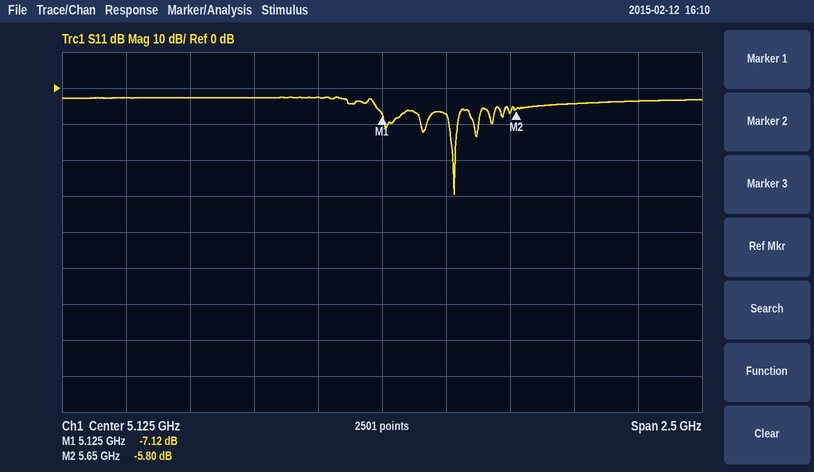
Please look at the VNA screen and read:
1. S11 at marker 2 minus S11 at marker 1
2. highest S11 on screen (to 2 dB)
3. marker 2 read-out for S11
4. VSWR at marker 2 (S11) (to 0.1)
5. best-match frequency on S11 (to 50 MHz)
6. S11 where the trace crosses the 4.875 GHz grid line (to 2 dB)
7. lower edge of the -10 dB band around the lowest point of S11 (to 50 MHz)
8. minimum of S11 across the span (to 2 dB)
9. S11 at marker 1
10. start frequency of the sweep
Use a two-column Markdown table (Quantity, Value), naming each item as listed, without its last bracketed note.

| Quantity | Value |
|---|---|
| S11 at marker 2 minus S11 at marker 1 | 1.32 dB |
| highest S11 on screen | -2 dB |
| marker 2 read-out for S11 | -5.80 dB |
| VSWR at marker 2 (S11) | 3.1 |
| best-match frequency on S11 | 5.40 GHz |
| S11 where the trace crosses the 4.875 GHz grid line | -2 dB |
| lower edge of the -10 dB band around the lowest point of S11 | 5.40 GHz |
| minimum of S11 across the span | -30 dB |
| S11 at marker 1 | -7.12 dB |
| start frequency of the sweep | 3.875 GHz |
